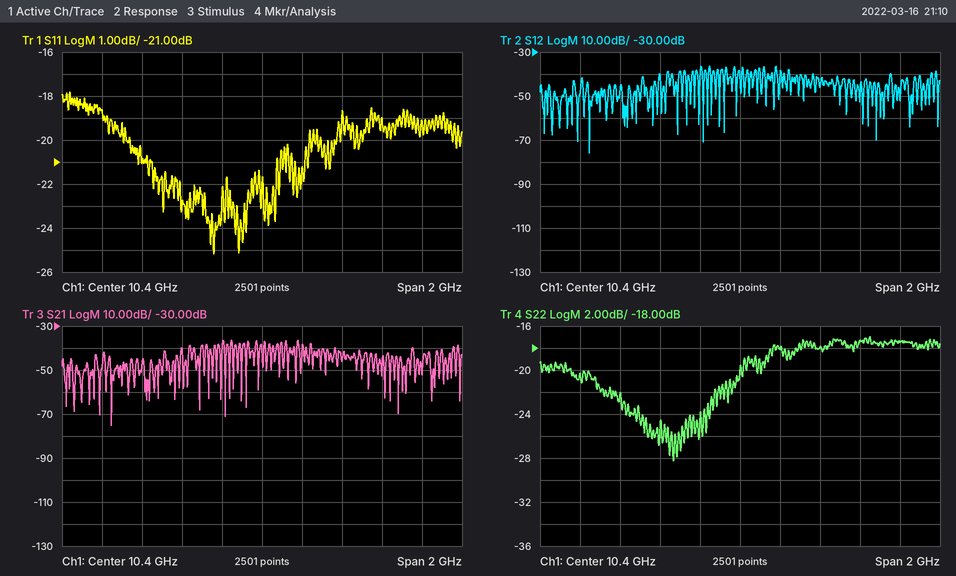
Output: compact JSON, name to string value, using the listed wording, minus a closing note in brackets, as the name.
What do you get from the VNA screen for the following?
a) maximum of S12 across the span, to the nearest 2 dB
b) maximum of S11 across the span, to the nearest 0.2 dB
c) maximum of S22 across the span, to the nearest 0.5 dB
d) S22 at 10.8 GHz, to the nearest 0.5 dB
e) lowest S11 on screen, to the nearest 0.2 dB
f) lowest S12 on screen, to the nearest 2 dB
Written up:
{"maximum of S12 across the span, to the nearest 2 dB": "-36 dB", "maximum of S11 across the span, to the nearest 0.2 dB": "-17.8 dB", "maximum of S22 across the span, to the nearest 0.5 dB": "-17.0 dB", "S22 at 10.8 GHz, to the nearest 0.5 dB": "-18.0 dB", "lowest S11 on screen, to the nearest 0.2 dB": "-25.2 dB", "lowest S12 on screen, to the nearest 2 dB": "-76 dB"}
